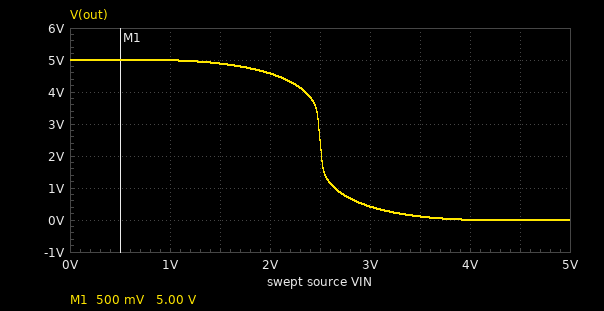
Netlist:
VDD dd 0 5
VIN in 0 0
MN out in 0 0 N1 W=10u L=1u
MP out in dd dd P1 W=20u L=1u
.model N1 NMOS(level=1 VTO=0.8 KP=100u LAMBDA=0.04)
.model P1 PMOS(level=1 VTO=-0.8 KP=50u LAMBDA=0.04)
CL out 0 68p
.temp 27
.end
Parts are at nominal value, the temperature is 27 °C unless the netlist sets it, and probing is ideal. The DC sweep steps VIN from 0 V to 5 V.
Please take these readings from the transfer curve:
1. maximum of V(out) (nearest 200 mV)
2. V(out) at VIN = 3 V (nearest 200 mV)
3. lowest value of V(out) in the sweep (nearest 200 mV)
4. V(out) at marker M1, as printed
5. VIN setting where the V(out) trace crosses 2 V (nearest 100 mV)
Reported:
5.0 V
400 mV
0 V
5.00 V
2.5 V
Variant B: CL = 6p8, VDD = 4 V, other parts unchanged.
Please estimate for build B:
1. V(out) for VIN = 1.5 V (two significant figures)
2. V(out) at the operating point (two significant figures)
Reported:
3.8 V
4.0 V
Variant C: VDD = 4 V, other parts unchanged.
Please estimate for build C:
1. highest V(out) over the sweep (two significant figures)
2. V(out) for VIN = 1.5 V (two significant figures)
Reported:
4.0 V
3.8 V
